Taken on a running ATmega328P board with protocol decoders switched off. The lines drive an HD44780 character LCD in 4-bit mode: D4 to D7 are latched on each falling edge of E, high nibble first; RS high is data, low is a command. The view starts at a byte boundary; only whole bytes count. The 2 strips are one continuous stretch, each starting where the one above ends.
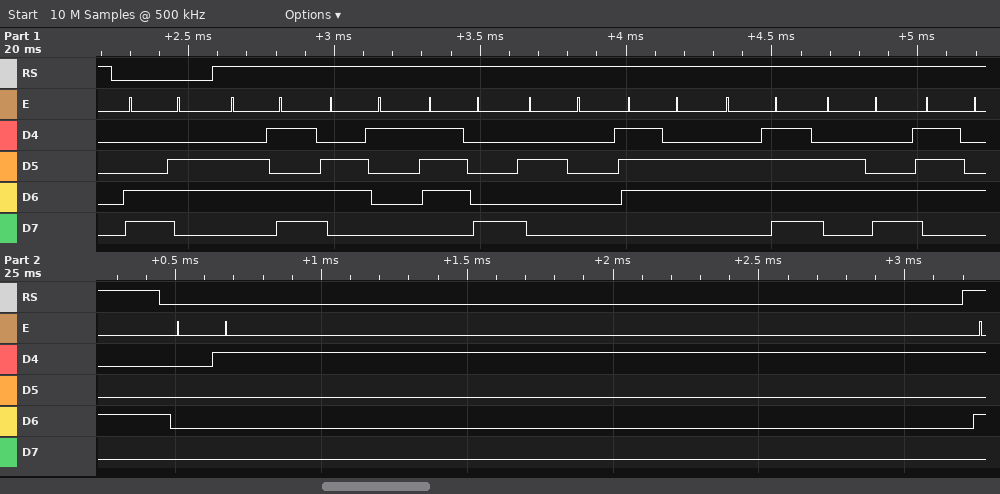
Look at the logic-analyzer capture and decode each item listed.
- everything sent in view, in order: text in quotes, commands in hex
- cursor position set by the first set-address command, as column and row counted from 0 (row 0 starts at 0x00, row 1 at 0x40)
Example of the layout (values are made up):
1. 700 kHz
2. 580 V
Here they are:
1. 0xC6 "max volt" 0x01
2. column 6, row 1
